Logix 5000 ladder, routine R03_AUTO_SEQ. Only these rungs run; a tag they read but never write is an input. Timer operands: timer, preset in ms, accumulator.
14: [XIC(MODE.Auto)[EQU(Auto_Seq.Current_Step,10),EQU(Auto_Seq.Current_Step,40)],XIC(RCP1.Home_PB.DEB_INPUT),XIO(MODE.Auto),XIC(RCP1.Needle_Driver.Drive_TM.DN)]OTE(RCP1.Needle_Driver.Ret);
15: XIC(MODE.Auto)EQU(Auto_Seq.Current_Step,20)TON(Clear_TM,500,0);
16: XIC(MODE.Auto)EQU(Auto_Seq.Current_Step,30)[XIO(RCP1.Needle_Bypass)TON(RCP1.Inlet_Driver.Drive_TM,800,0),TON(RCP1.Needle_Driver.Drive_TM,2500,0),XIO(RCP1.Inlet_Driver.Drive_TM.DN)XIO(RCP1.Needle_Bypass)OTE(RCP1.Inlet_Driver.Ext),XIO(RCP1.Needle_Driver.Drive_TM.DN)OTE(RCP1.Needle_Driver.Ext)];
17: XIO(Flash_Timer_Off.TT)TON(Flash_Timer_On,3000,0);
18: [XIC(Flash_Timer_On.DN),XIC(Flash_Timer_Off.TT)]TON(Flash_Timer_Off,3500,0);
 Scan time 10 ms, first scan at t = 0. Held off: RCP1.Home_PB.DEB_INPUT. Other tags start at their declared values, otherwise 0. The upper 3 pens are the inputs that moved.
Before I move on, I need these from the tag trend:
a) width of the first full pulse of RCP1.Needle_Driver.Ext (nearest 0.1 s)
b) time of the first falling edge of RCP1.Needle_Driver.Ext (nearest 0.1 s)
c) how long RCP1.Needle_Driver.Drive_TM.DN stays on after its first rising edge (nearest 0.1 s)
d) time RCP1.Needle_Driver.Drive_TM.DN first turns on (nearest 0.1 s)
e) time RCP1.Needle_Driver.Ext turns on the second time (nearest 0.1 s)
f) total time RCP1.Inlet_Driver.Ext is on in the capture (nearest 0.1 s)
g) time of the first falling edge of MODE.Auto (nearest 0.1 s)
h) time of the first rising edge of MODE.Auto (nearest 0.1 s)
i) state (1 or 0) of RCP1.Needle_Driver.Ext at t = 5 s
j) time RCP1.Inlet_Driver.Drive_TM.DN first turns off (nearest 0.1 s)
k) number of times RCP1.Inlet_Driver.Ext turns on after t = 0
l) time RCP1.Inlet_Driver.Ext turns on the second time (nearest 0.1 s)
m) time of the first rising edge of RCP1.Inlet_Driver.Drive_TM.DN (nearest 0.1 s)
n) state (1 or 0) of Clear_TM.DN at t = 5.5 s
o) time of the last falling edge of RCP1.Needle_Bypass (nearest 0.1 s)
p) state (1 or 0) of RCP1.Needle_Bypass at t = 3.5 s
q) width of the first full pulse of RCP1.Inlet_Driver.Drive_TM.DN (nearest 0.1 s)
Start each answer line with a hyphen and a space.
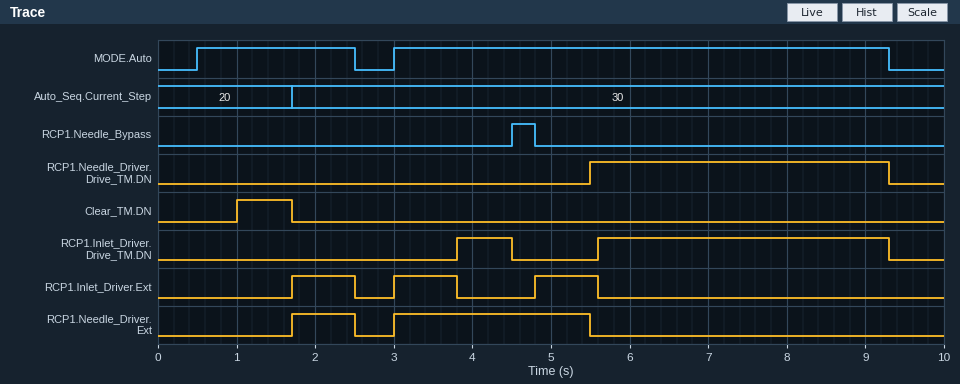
- 0.8 s
- 2.5 s
- 3.8 s
- 5.5 s
- 3.0 s
- 2.4 s
- 2.5 s
- 0.5 s
- 1
- 4.5 s
- 3
- 3.0 s
- 3.8 s
- 0
- 4.8 s
- 0
- 0.7 s
